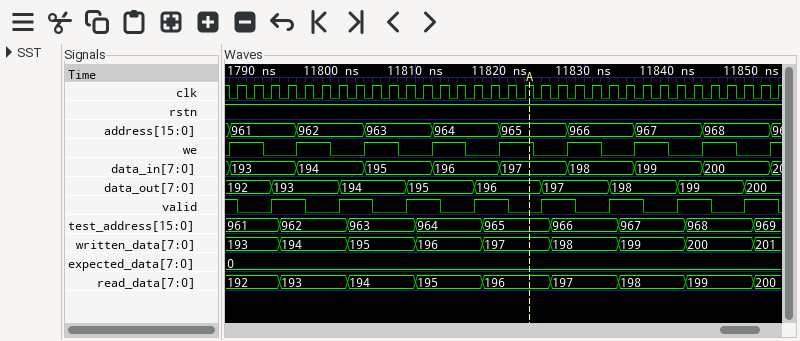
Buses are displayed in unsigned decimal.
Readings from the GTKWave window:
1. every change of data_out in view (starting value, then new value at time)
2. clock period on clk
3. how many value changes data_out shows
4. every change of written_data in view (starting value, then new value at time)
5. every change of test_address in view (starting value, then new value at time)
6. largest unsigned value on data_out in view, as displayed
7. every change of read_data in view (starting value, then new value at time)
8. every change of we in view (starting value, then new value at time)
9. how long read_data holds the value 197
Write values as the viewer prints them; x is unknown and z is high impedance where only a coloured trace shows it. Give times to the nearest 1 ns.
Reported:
192, 193 at 11793 ns, 194 at 11801 ns, 195 at 11809 ns, 196 at 11817 ns, 197 at 11825 ns, 198 at 11833 ns, 199 at 11841 ns, 200 at 11849 ns
2 ns
8
193, 194 at 11794 ns, 195 at 11802 ns, 196 at 11810 ns, 197 at 11818 ns, 198 at 11826 ns, 199 at 11834 ns, 200 at 11842 ns, 201 at 11850 ns
961, 962 at 11794 ns, 963 at 11802 ns, 964 at 11810 ns, 965 at 11818 ns, 966 at 11826 ns, 967 at 11834 ns, 968 at 11842 ns, 969 at 11850 ns
200
192, 193 at 11794 ns, 194 at 11802 ns, 195 at 11810 ns, 196 at 11818 ns, 197 at 11826 ns, 198 at 11834 ns, 199 at 11842 ns, 200 at 11850 ns
0, 1 at 11788 ns, 0 at 11792 ns, 1 at 11796 ns, 0 at 11800 ns, 1 at 11804 ns, 0 at 11808 ns, 1 at 11812 ns, 0 at 11816 ns, 1 at 11820 ns, 0 at 11824 ns, 1 at 11828 ns, 0 at 11832 ns, 1 at 11836 ns, 0 at 11840 ns, 1 at 11844 ns, 0 at 11848 ns, 1 at 11852 ns
8 ns
